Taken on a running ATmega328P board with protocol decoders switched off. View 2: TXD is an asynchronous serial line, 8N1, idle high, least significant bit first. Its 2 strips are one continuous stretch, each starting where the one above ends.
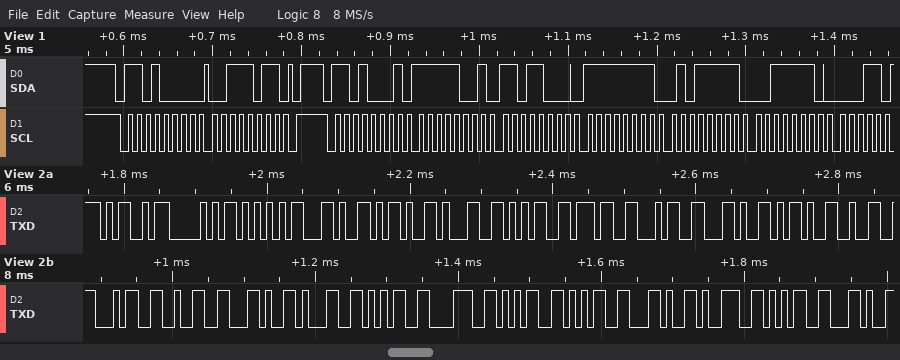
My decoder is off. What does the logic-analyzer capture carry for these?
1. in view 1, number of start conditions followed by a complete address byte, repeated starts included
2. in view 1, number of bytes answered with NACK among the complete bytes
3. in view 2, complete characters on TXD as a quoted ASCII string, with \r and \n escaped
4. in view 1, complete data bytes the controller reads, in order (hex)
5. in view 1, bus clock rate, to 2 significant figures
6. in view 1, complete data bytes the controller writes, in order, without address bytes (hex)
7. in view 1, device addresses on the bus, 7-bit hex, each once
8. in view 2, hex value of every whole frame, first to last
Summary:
2
0
"MPU,-1574,-242,15855,95,"
F9 D8 FF 5F 3E
100 kHz
3B
0x68
4D 50 55 2C 2D 31 35 37 34 2C 2D 32 34 32 2C 31 35 38 35 35 2C 39 35 2C
